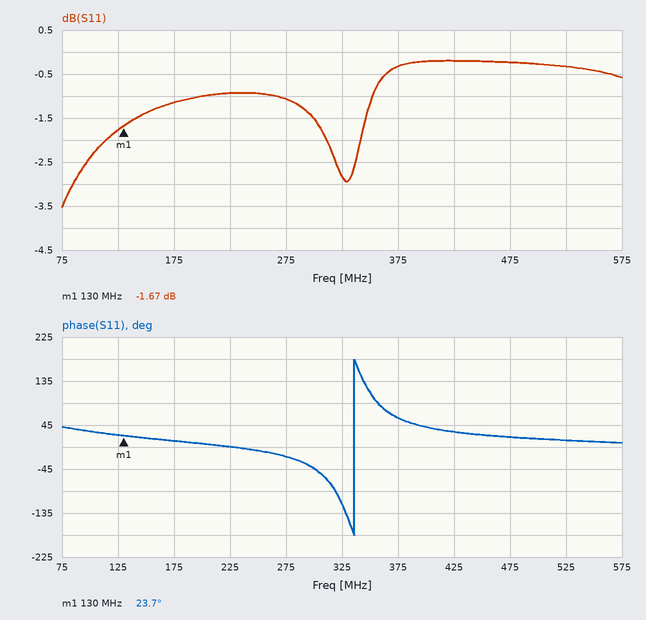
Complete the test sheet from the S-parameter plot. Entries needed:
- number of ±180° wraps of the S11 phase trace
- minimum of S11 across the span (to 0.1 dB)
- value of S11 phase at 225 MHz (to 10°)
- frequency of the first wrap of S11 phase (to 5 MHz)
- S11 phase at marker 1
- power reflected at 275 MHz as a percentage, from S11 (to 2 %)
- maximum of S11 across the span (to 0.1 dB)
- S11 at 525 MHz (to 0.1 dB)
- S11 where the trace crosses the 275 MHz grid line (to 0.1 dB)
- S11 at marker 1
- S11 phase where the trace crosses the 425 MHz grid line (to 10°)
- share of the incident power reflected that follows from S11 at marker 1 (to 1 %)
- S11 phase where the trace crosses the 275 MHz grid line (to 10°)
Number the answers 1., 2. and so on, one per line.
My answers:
1. 1
2. -3.5 dB
3. 0°
4. 335 MHz
5. 23.7°
6. 78 %
7. -0.2 dB
8. -0.3 dB
9. -1.1 dB
10. -1.67 dB
11. 30°
12. 68 %
13. -20°
